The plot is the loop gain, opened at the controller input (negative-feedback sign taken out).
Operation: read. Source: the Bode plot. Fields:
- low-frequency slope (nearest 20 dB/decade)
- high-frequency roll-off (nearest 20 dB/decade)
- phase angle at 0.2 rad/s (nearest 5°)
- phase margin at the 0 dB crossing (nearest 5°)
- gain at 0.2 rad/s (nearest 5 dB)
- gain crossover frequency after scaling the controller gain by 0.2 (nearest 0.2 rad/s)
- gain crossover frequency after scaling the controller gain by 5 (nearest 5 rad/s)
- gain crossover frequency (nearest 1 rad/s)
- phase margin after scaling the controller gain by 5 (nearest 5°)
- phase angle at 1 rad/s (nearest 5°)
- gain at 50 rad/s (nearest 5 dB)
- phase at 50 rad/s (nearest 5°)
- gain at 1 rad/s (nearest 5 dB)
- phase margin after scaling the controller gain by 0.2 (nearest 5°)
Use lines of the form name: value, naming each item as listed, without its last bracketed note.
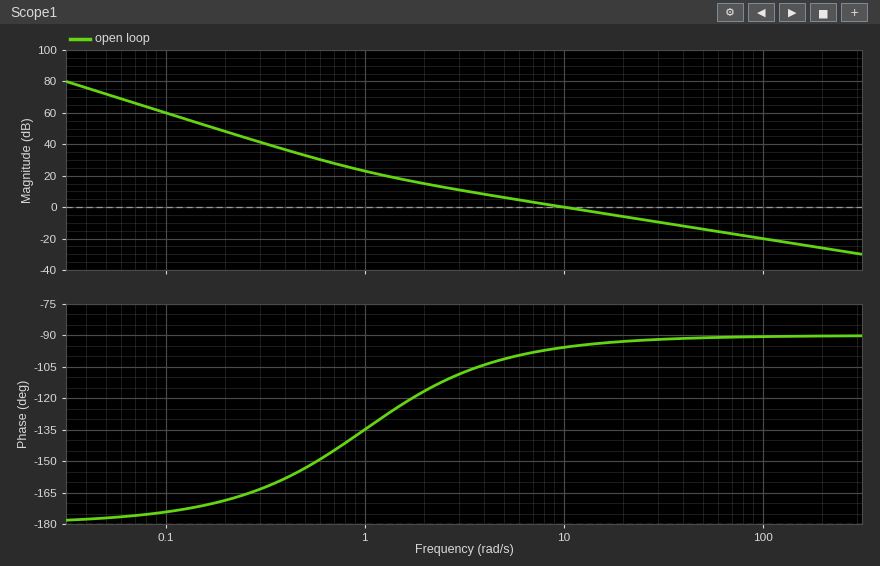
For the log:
low-frequency slope: -40 dB/decade
high-frequency roll-off: -20 dB/decade
phase angle at 0.2 rad/s: -170°
phase margin at the 0 dB crossing: 85°
gain at 0.2 rad/s: 50 dB
gain crossover frequency after scaling the controller gain by 0.2: 2.2 rad/s
gain crossover frequency after scaling the controller gain by 5: 50 rad/s
gain crossover frequency: 10 rad/s
phase margin after scaling the controller gain by 5: 90°
phase angle at 1 rad/s: -135°
gain at 50 rad/s: -15 dB
phase at 50 rad/s: -90°
gain at 1 rad/s: 25 dB
phase margin after scaling the controller gain by 0.2: 65°
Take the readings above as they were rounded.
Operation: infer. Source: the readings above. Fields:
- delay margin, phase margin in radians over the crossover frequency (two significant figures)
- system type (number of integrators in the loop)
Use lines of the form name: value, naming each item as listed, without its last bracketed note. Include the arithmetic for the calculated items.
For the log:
delay margin, phase margin in radians over the crossover frequency: 85 × π / 180 / 10 = 0.15 s
system type: 2
